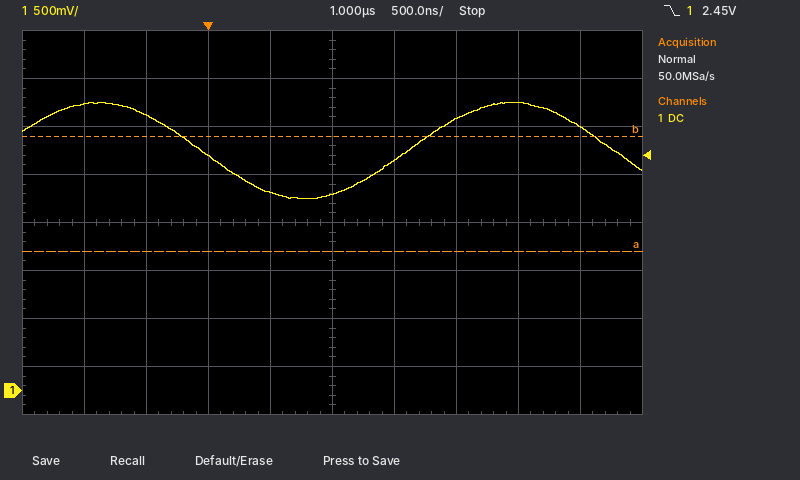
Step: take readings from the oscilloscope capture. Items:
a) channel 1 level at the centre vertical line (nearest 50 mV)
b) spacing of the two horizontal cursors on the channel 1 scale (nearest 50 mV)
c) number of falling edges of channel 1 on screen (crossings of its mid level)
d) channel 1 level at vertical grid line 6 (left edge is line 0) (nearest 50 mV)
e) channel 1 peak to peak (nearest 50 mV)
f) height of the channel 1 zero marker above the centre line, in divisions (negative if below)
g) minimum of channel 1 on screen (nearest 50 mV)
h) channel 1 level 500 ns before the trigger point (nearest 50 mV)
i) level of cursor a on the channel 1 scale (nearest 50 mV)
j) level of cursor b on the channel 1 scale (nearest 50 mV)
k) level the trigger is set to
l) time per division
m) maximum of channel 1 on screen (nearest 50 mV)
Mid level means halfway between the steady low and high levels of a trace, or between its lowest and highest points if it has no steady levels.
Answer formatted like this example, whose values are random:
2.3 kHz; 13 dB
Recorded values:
2.05 V; 1.20 V; 2; 2.40 V; 1.00 V; -3.5 div; 2.00 V; 2.85 V; 1.45 V; 2.65 V; 2.45 V; 500 ns; 3.00 V
